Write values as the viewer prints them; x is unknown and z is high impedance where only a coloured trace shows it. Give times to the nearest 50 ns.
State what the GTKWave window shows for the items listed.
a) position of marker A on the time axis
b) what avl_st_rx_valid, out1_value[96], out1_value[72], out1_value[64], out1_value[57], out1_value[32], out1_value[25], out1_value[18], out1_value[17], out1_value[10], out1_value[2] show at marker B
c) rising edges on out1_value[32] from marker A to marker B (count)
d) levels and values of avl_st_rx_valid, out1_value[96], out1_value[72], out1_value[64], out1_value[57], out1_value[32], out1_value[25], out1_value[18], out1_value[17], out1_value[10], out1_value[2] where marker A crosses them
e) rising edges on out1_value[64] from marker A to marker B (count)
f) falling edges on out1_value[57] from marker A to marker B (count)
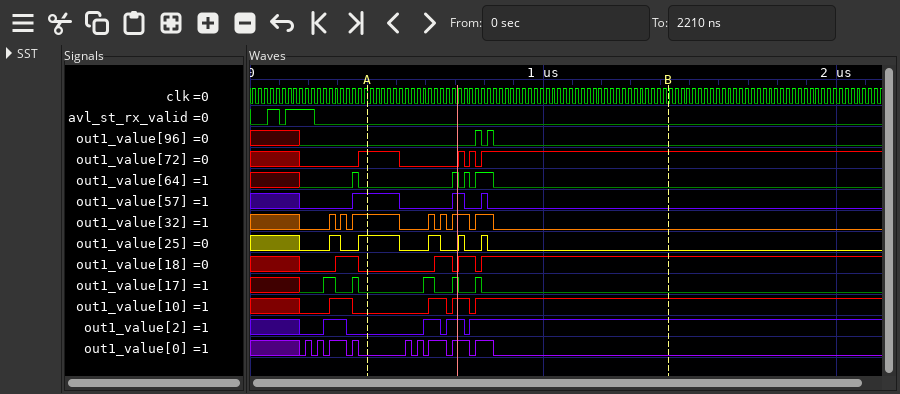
400 ns
avl_st_rx_valid=0, out1_value[96]=0, out1_value[72]=1, out1_value[64]=0, out1_value[57]=0, out1_value[32]=0, out1_value[25]=0, out1_value[18]=1, out1_value[17]=0, out1_value[10]=1, out1_value[2]=1
4
avl_st_rx_valid=0, out1_value[96]=0, out1_value[72]=1, out1_value[64]=0, out1_value[57]=1, out1_value[32]=1, out1_value[25]=1, out1_value[18]=0, out1_value[17]=0, out1_value[10]=0, out1_value[2]=0
3
3
